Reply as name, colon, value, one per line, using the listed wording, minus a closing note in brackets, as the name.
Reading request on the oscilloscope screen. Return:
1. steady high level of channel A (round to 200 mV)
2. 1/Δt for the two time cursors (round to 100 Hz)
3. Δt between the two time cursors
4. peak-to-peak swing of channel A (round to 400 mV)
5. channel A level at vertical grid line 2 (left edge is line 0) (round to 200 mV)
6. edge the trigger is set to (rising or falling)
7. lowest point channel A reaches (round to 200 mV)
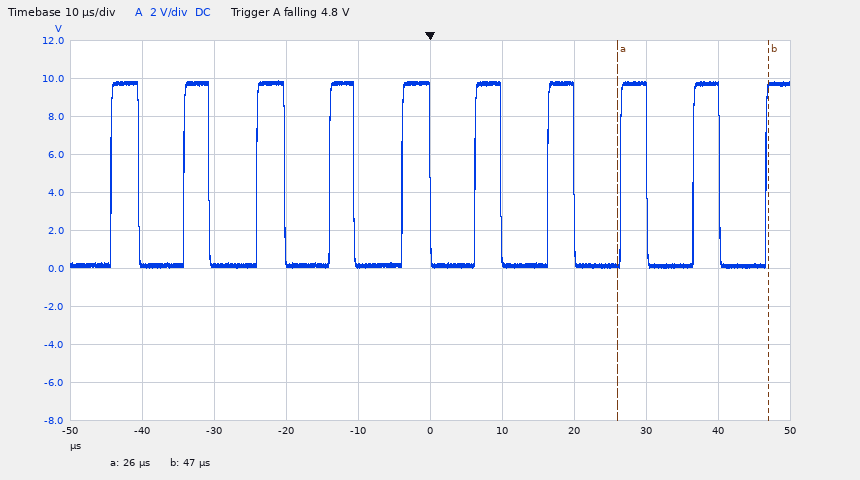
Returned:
steady high level of channel A: 9.8 V
1/Δt for the two time cursors: 47.6 kHz
Δt between the two time cursors: 21 µs
peak-to-peak swing of channel A: 10.0 V
channel A level at vertical grid line 2 (left edge is line 0): 200 mV
edge the trigger is set to: falling
lowest point channel A reaches: 0.0 V
